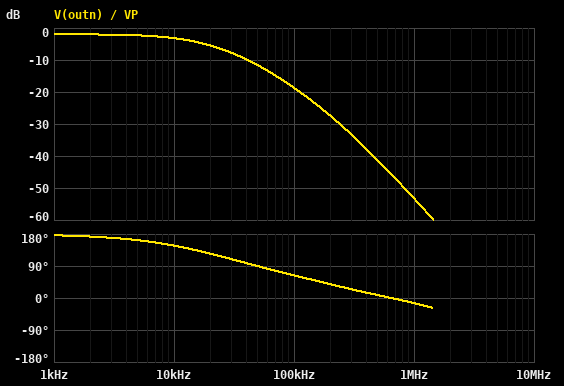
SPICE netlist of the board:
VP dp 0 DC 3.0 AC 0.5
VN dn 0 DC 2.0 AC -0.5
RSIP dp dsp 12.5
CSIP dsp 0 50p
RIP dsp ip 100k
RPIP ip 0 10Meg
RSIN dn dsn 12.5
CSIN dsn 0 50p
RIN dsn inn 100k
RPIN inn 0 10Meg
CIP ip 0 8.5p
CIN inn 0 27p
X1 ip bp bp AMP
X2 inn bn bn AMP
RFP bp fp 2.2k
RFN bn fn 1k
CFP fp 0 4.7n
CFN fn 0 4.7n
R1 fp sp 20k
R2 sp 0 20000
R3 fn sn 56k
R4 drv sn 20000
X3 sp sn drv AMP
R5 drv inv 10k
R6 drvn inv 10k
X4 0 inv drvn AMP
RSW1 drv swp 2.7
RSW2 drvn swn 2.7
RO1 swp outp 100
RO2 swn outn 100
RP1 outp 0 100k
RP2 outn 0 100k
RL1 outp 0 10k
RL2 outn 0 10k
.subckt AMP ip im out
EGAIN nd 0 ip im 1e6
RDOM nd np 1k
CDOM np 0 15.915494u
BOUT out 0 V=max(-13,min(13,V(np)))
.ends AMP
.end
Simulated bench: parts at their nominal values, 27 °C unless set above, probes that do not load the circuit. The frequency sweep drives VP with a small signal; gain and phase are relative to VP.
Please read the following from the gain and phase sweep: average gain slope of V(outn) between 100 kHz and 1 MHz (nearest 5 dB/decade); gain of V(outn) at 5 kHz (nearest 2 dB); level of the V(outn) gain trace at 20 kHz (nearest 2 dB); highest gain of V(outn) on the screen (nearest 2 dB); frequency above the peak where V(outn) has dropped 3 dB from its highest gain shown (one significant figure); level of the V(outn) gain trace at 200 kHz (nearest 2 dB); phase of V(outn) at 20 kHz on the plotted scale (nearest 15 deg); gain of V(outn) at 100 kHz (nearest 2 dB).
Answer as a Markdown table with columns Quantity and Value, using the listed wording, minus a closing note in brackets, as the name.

| Quantity | Value |
|---|---|
| average gain slope of V(outn) between 100 kHz and 1 MHz | -35 dB/decade |
| gain of V(outn) at 5 kHz | -2 dB |
| level of the V(outn) gain trace at 20 kHz | -6 dB |
| highest gain of V(outn) on the screen | -2 dB |
| frequency above the peak where V(outn) has dropped 3 dB from its highest gain shown | 20 kHz |
| level of the V(outn) gain trace at 200 kHz | -28 dB |
| phase of V(outn) at 20 kHz on the plotted scale | 120 deg |
| gain of V(outn) at 100 kHz | -18 dB |
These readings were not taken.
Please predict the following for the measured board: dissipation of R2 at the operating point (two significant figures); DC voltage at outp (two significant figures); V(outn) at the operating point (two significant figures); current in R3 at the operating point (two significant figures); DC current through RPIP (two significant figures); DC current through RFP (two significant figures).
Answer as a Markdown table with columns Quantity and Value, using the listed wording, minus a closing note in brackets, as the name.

| Quantity | Value |
|---|---|
| dissipation of R2 at the operating point | 99 µW |
| DC voltage at outp | 1.2 V |
| V(outn) at the operating point | -1.2 V |
| current in R3 at the operating point | 10 µA |
| DC current through RPIP | 300 nA |
| DC current through RFP | 70 µA |
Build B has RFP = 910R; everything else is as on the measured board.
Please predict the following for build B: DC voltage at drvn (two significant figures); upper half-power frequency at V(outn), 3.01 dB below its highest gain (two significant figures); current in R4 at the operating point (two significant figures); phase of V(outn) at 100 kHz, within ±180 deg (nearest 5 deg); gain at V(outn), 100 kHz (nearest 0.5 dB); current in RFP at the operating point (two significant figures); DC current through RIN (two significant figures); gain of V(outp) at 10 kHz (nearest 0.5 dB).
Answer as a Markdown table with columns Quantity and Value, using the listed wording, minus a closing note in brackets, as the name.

| Quantity | Value |
|---|---|
| DC voltage at drvn | -1.3 V |
| upper half-power frequency at V(outn), 3.01 dB below its highest gain | 34 kHz |
| current in R4 at the operating point | 9.3 µA |
| phase of V(outn) at 100 kHz, within ±180 deg | 75 deg |
| gain at V(outn), 100 kHz | -13.0 dB |
| current in RFP at the operating point | 73 µA |
| DC current through RIN | 200 nA |
| gain of V(outp) at 10 kHz | -2.0 dB |
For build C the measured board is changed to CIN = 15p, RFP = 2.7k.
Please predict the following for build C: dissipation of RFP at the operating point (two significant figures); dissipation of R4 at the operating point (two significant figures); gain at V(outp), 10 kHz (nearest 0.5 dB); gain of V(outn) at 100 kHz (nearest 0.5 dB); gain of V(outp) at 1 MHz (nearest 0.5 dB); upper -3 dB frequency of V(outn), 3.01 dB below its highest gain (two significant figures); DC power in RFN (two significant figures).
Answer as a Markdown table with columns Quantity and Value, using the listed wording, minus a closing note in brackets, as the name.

| Quantity | Value |
|---|---|
| dissipation of RFP at the operating point | 13 µW |
| dissipation of R4 at the operating point | 2.1 µW |
| gain at V(outp), 10 kHz | -3.5 dB |
| gain of V(outn) at 100 kHz | -19.0 dB |
| gain of V(outp) at 1 MHz | -53.5 dB |
| upper -3 dB frequency of V(outn), 3.01 dB below its highest gain | 15 kHz |
| DC power in RFN | 110 nW |
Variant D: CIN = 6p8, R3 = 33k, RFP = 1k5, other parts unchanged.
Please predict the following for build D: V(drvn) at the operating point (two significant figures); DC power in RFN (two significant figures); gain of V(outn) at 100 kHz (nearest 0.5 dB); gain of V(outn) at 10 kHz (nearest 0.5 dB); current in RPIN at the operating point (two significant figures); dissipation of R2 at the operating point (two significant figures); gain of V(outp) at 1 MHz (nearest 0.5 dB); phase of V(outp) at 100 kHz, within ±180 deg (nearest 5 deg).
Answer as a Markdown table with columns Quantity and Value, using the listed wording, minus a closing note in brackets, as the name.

| Quantity | Value |
|---|---|
| V(drvn) at the operating point | -1.1 V |
| DC power in RFN | 260 nW |
| gain of V(outn) at 100 kHz | -12.5 dB |
| gain of V(outn) at 10 kHz | -0.5 dB |
| current in RPIN at the operating point | 200 nA |
| dissipation of R2 at the operating point | 100 µW |
| gain of V(outp) at 1 MHz | -45.0 dB |
| phase of V(outp) at 100 kHz, within ±180 deg | -100 deg |
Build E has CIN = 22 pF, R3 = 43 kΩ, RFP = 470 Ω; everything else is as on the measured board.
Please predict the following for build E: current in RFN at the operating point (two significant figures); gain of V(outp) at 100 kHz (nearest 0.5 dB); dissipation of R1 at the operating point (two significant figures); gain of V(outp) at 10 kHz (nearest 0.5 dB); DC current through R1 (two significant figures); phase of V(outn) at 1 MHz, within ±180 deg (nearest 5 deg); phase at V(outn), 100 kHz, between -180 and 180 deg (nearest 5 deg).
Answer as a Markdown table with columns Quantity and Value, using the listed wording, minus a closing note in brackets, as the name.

| Quantity | Value |
|---|---|
| current in RFN at the operating point | 12 µA |
| gain of V(outp) at 100 kHz | -8.0 dB |
| dissipation of R1 at the operating point | 110 µW |
| gain of V(outp) at 10 kHz | -1.0 dB |
| DC current through R1 | 73 µA |
| phase of V(outn) at 1 MHz, within ±180 deg | -10 deg |
| phase at V(outn), 100 kHz, between -180 and 180 deg | 90 deg |
